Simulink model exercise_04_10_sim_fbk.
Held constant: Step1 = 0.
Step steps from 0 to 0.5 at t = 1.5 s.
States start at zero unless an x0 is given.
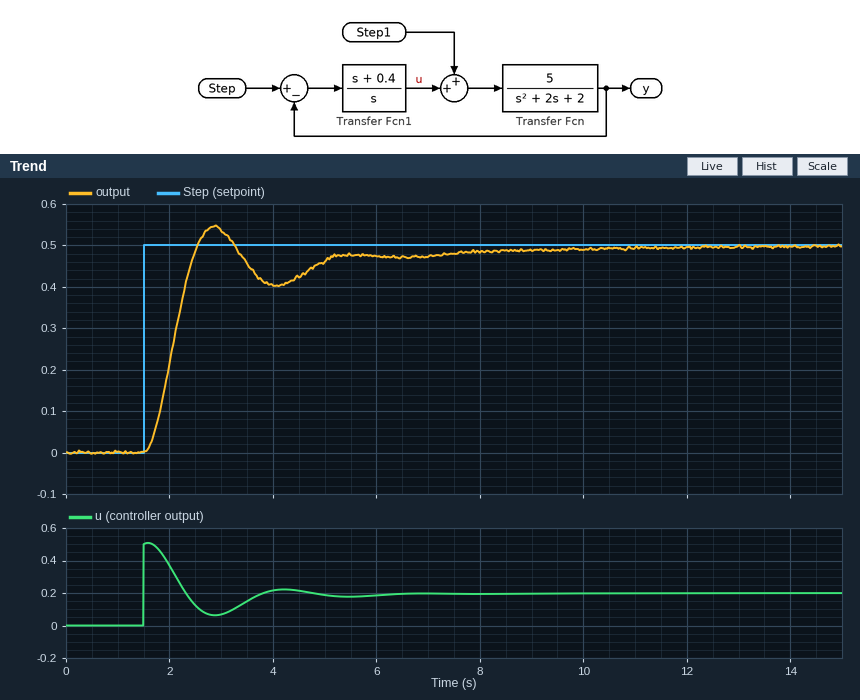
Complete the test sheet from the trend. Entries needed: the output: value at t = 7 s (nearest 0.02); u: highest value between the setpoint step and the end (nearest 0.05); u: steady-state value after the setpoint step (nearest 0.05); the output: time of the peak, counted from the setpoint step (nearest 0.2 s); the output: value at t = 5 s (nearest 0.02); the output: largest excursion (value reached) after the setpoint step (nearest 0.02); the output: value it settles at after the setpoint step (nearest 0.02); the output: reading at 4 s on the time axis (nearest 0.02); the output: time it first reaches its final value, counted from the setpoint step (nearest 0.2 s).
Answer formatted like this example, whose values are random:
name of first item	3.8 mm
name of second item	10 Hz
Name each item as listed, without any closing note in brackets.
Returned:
the output: value at t = 7 s	0.48
u: highest value between the setpoint step and the end	0.50
u: steady-state value after the setpoint step	0.20
the output: time of the peak, counted from the setpoint step	1.4 s
the output: value at t = 5 s	0.46
the output: largest excursion (value reached) after the setpoint step	0.54
the output: value it settles at after the setpoint step	0.50
the output: reading at 4 s on the time axis	0.40
the output: time it first reaches its final value, counted from the setpoint step	1.0 s
